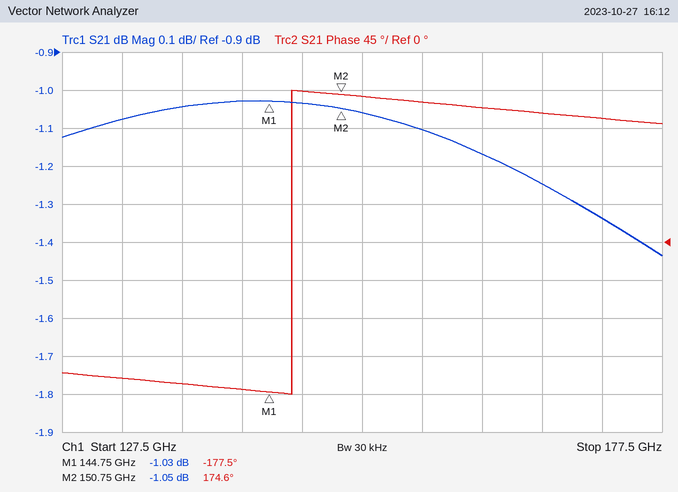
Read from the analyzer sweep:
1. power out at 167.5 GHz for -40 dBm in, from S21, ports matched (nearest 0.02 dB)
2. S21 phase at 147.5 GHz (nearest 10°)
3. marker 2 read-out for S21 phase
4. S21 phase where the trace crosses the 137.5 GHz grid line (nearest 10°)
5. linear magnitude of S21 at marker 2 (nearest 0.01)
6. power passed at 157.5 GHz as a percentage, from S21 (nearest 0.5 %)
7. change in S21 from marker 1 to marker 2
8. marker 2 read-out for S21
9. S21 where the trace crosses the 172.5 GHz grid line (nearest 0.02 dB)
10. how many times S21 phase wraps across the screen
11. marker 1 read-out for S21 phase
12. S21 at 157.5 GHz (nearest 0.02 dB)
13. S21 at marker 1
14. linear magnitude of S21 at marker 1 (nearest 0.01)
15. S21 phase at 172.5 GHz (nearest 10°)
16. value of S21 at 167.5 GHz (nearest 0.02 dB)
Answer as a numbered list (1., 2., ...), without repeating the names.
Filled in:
1. -41.24 dBm
2. 180°
3. 174.6°
4. -170°
5. 0.89
6. 77.5 %
7. -0.02 dB
8. -1.05 dB
9. -1.34 dB
10. 1
11. -177.5°
12. -1.10 dB
13. -1.03 dB
14. 0.89
15. 150°
16. -1.24 dB
